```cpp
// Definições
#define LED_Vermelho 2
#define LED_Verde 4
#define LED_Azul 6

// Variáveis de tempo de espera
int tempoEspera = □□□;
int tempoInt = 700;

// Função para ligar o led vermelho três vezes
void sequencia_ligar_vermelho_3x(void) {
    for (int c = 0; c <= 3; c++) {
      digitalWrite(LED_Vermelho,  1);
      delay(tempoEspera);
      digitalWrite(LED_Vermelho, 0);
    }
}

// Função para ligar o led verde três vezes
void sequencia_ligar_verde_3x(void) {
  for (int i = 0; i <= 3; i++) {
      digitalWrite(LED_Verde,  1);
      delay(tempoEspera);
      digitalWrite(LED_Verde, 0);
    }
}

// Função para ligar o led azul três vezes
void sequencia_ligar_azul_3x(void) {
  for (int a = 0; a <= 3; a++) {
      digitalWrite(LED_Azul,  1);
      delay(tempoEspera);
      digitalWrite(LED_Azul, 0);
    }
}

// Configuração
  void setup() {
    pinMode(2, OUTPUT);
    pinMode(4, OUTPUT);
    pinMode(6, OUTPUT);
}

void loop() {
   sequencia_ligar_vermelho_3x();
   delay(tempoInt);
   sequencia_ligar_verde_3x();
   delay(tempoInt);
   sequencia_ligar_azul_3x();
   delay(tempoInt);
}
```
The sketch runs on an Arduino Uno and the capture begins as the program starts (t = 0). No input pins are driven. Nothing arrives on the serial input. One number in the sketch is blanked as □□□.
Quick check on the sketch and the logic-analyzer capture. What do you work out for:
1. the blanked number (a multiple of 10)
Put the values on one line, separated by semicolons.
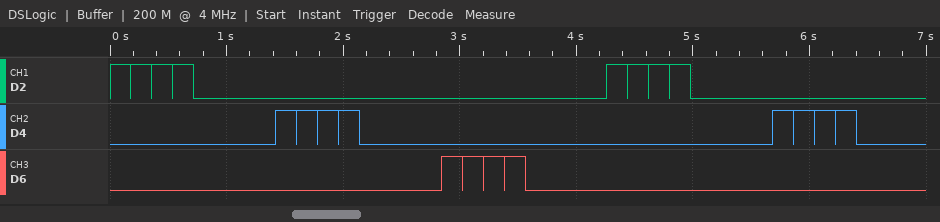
180
